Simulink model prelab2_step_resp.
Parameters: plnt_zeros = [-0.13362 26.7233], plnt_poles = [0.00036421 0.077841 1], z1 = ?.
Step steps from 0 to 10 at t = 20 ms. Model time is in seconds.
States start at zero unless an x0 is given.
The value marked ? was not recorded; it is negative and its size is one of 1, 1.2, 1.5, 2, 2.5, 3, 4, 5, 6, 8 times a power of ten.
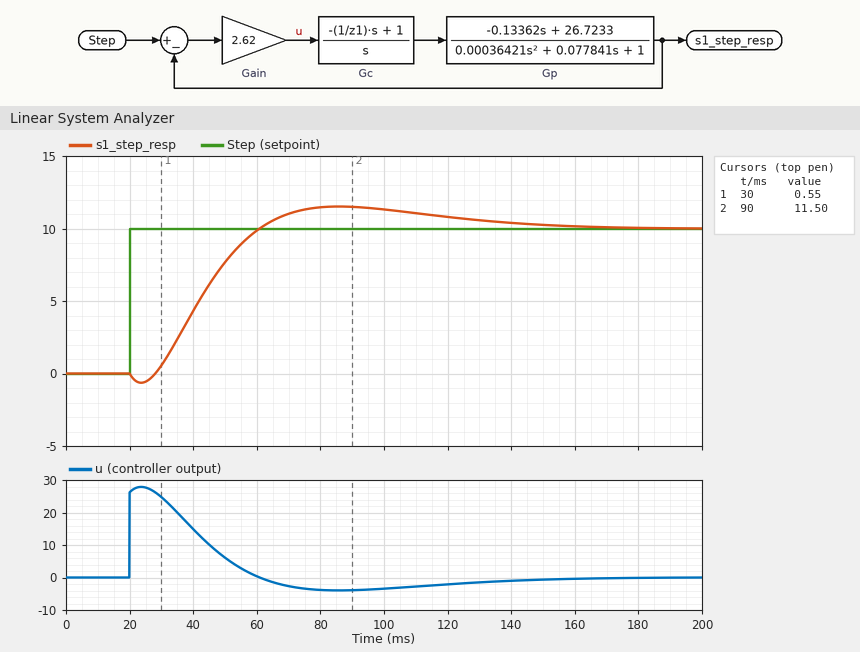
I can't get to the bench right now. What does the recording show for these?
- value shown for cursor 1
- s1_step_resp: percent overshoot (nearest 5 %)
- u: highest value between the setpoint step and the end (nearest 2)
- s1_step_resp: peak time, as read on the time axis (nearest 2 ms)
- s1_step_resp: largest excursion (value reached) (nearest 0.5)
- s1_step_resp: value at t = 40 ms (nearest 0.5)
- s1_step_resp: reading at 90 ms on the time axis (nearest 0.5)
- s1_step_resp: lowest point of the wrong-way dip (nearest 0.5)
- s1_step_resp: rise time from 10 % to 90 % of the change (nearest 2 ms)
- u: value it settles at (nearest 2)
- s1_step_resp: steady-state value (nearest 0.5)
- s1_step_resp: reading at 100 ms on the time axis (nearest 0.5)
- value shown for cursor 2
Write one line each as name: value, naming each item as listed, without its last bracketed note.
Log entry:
value shown for cursor 1: 0.55
s1_step_resp: percent overshoot: 15 %
u: highest value between the setpoint step and the end: 28
s1_step_resp: peak time, as read on the time axis: 86 ms
s1_step_resp: largest excursion (value reached): 11.5
s1_step_resp: value at t = 40 ms: 4.5
s1_step_resp: reading at 90 ms on the time axis: 11.5
s1_step_resp: lowest point of the wrong-way dip: -0.5
s1_step_resp: rise time from 10 % to 90 % of the change: 24 ms
u: value it settles at: 0
s1_step_resp: steady-state value: 10.0
s1_step_resp: reading at 100 ms on the time axis: 11.5
value shown for cursor 2: 11.50
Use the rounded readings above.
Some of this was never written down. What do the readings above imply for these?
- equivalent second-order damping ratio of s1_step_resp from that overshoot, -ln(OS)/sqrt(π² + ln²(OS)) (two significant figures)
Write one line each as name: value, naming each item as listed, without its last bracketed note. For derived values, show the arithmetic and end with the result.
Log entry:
equivalent second-order damping ratio of s1_step_resp from that overshoot, -ln(OS)/sqrt(π² + ln²(OS)): ln(0.15) = -1.897; 1.897 / sqrt(9.870 + 3.599) = 0.52
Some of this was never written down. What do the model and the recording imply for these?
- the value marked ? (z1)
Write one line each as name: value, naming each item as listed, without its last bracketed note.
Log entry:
the value marked ?: -25
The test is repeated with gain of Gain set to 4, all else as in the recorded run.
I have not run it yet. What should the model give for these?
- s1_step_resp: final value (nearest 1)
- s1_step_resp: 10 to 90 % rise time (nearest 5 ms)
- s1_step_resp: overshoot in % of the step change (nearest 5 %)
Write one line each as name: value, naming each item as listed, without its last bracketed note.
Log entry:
s1_step_resp: final value: 10
s1_step_resp: 10 to 90 % rise time: 15 ms
s1_step_resp: overshoot in % of the step change: 25 %
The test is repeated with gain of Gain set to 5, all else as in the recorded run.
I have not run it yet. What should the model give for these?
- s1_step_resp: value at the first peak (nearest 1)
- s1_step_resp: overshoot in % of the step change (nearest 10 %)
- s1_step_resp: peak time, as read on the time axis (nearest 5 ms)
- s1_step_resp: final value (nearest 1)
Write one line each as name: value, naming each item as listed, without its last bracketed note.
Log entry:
s1_step_resp: value at the first peak: 13
s1_step_resp: overshoot in % of the step change: 30 %
s1_step_resp: peak time, as read on the time axis: 55 ms
s1_step_resp: final value: 10
